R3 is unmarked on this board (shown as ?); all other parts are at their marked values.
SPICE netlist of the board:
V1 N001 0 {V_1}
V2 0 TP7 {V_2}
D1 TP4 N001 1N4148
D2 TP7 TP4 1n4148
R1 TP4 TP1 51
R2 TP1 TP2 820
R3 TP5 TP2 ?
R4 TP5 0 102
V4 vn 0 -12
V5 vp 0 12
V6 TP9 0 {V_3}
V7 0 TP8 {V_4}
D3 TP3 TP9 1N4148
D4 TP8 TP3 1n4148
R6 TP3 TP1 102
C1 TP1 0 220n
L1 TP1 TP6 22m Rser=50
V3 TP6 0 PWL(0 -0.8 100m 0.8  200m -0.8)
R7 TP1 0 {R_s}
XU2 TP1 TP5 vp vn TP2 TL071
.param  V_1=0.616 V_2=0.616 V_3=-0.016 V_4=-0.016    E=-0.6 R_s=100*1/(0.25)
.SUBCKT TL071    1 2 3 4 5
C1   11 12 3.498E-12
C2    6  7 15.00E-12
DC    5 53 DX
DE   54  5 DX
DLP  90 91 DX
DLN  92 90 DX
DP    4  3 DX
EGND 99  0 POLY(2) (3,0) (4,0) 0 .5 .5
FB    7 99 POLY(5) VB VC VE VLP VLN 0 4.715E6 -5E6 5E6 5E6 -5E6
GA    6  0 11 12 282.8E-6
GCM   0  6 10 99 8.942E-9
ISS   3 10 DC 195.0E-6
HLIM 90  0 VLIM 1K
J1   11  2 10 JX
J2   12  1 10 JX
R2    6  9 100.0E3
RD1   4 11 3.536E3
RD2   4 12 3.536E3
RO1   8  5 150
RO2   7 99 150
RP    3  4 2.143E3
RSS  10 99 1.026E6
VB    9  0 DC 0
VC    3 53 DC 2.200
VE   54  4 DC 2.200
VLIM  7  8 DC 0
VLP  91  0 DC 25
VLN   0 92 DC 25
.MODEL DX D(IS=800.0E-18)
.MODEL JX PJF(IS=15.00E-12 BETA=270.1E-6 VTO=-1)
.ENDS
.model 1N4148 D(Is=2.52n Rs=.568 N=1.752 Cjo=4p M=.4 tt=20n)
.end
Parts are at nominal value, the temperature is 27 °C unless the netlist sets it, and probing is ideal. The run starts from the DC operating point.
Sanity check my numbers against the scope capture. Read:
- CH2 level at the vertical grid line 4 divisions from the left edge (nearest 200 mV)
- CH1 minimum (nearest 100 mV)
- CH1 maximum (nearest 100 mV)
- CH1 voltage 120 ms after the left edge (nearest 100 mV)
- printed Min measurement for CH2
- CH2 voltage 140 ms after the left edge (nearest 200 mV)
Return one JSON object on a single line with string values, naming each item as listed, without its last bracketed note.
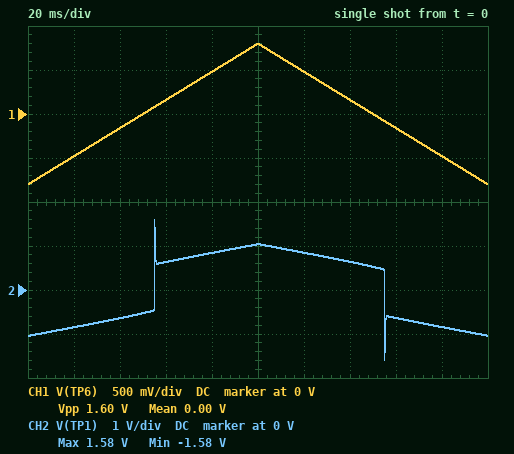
{"CH2 level at the vertical grid line 4 divisions from the left edge": "800 mV", "CH1 minimum": "-800 mV", "CH1 maximum": "800 mV", "CH1 voltage 120 ms after the left edge": "500 mV", "printed Min measurement for CH2": "-1.58 V", "CH2 voltage 140 ms after the left edge": "600 mV"}
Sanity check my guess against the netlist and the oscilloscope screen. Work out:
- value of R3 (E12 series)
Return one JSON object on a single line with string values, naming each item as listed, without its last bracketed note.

{"value of R3": "2.2 kΩ"}
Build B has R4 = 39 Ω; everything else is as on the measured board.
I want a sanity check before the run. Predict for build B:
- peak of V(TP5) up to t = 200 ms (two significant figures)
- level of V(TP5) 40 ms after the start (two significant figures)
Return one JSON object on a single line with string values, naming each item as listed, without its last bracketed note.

{"peak of V(TP5) up to t = 200 ms": "180 mV", "level of V(TP5) 40 ms after the start": "-180 mV"}
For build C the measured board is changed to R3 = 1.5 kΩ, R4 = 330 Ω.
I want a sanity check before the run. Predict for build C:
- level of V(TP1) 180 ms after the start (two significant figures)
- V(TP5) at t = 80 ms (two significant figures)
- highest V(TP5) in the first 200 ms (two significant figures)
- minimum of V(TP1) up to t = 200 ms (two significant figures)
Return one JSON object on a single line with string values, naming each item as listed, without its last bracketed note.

{"level of V(TP1) 180 ms after the start": "-550 mV", "V(TP5) at t = 80 ms": "550 mV", "highest V(TP5) in the first 200 ms": "1.1 V", "minimum of V(TP1) up to t = 200 ms": "-1.1 V"}
